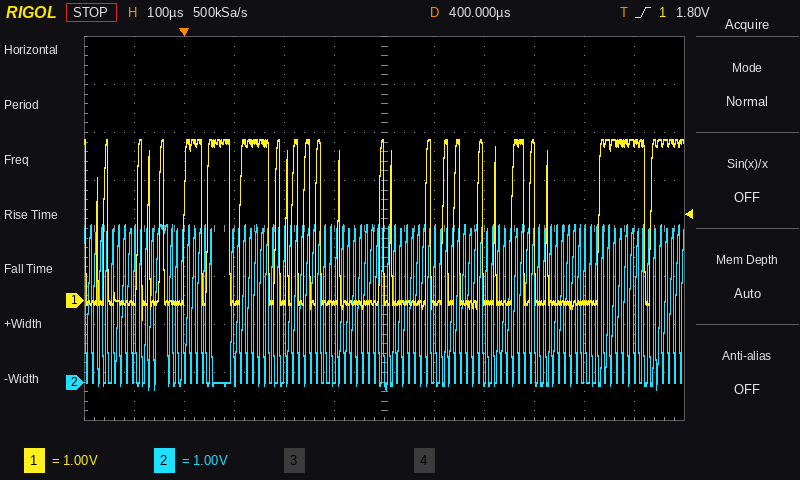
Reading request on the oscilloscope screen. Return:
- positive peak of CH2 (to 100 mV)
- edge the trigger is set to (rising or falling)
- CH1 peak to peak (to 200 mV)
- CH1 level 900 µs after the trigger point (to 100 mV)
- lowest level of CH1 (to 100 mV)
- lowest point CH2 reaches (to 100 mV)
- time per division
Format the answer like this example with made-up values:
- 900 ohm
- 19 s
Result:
- 3.3 V
- rising
- 3.8 V
- 3.3 V
- -400 mV
- -200 mV
- 100 µs
